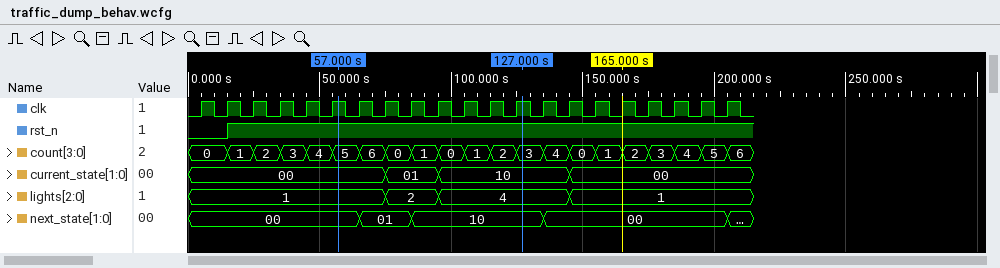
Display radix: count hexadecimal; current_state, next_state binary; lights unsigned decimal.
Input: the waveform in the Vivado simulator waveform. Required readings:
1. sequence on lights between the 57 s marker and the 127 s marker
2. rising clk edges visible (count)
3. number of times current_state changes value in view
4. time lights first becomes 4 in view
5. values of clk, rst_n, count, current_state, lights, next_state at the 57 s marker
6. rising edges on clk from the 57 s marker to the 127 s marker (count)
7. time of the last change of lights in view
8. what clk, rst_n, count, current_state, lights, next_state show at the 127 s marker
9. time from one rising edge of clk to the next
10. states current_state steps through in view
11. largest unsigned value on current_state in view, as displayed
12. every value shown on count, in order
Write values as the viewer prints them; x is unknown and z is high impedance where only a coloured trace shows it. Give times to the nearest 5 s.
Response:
1, 2, 4
21
3
95 s
clk=1, rst_n=1, count=5, current_state=00, lights=1, next_state=00
7
145 s
clk=1, rst_n=1, count=3, current_state=10, lights=4, next_state=10
10 s
00, 01, 10, 00
10
0, 1, 2, 3, 4, 5, 6, 0, 1, 0, 1, 2, 3, 4, 0, 1, 2, 3, 4, 5, 6
